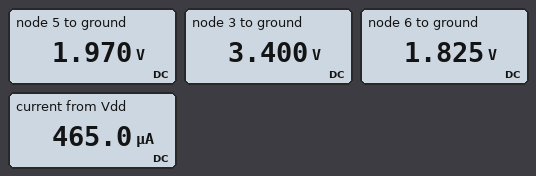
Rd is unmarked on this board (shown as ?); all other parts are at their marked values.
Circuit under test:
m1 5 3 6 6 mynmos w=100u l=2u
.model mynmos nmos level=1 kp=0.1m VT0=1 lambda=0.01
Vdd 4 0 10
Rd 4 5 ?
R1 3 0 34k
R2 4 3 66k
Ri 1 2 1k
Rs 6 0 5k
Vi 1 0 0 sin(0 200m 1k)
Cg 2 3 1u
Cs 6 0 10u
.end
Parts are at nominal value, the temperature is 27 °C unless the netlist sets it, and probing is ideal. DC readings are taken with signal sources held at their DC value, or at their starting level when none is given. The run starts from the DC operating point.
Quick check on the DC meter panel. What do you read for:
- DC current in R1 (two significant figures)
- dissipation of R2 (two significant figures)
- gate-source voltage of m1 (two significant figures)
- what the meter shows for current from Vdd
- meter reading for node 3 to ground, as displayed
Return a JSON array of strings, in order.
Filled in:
["100 µA", "660 µW", "1.6 V", "465.0 µA", "3.400 V"]
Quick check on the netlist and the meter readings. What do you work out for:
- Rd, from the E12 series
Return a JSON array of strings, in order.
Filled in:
["22 kΩ"]
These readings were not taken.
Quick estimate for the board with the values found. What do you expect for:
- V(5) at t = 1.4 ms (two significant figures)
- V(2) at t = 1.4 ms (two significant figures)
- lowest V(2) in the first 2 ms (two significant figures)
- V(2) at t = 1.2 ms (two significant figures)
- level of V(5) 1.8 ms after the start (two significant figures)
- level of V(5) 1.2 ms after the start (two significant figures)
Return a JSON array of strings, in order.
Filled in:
["1.9 V", "110 mV", "-190 mV", "180 mV", "2.1 V", "1.9 V"]
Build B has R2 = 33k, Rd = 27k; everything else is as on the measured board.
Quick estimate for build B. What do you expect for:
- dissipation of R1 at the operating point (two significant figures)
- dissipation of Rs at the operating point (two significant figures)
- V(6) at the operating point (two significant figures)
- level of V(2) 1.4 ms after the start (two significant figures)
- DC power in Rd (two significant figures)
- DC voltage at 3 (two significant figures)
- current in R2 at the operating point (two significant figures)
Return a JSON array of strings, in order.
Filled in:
["760 µW", "490 µW", "1.6 V", "110 mV", "2.6 mW", "5.1 V", "150 µA"]
